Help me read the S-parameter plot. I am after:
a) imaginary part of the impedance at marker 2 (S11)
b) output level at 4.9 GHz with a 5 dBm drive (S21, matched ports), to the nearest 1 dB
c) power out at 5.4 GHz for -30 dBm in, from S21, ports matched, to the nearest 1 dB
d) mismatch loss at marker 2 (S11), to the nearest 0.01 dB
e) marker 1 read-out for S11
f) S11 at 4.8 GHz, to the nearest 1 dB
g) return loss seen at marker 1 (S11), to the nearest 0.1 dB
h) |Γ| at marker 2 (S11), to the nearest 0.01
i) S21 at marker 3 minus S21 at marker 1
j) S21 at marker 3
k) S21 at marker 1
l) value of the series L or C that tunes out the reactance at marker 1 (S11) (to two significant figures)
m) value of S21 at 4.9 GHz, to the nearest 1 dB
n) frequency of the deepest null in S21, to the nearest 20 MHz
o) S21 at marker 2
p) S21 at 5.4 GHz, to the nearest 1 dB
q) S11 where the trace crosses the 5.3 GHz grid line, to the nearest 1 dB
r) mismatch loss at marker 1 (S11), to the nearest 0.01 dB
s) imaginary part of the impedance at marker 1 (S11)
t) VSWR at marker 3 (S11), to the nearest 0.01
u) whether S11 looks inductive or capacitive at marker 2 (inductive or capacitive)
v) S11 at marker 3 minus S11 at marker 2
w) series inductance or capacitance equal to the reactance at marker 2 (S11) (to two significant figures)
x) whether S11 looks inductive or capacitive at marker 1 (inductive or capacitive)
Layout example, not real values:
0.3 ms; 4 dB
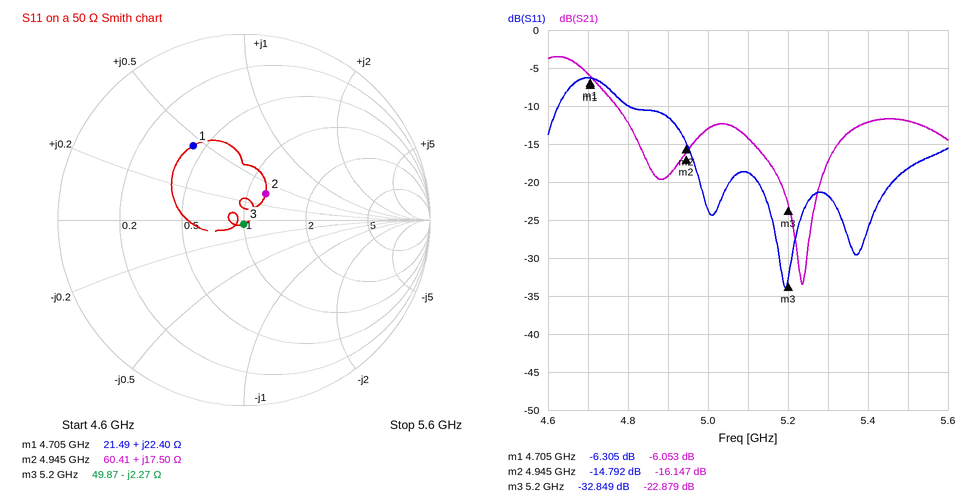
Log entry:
+17.50 Ω; -14 dBm; -42 dBm; 0.15 dB; -6.305 dB; -10 dB; 6.3 dB; 0.18; -16.826 dB; -22.879 dB; -6.053 dB; 1.5 pF; -19 dB; 5.24 GHz; -16.147 dB; -12 dB; -22 dB; 1.16 dB; +22.40 Ω; 1.05; inductive; -18.057 dB; 560 pH; inductive
